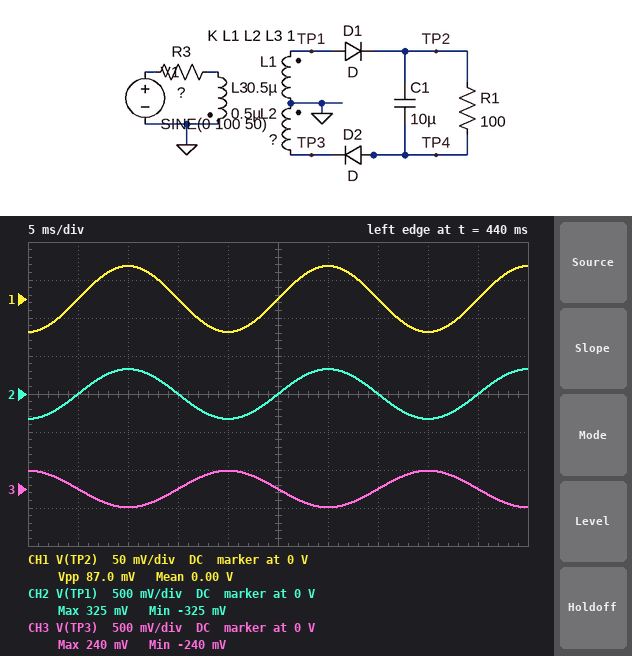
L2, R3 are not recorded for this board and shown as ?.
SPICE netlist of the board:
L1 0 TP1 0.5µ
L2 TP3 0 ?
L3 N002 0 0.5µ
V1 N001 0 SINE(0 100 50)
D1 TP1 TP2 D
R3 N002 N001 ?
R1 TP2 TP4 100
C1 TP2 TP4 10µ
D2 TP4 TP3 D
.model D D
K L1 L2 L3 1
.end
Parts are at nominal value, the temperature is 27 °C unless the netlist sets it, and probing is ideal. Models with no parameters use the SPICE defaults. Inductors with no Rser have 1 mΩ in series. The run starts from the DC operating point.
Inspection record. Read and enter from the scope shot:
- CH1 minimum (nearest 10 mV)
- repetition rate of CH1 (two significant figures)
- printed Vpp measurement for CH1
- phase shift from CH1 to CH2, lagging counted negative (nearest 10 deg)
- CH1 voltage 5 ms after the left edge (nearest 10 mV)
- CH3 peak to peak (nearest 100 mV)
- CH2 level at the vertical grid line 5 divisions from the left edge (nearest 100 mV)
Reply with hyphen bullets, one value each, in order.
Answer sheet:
- -40 mV
- 50 Hz
- 87.0 mV
- 0 deg
- 0 V
- 500 mV
- 0 V
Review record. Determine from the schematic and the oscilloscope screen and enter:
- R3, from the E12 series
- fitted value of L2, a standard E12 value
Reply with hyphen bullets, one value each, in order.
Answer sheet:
- 0.047 Ω
- 270 nH
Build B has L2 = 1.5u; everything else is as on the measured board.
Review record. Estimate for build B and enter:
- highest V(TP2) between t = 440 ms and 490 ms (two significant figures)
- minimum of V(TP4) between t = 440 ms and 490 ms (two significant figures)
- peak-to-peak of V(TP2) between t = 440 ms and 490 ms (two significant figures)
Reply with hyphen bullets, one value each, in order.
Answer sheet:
- 120 mV
- -120 mV
- 240 mV
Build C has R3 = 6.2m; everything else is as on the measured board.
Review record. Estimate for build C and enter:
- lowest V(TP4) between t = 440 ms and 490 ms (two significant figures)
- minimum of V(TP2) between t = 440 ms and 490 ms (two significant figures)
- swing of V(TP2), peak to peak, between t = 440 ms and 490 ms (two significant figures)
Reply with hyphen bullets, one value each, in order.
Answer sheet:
- -870 mV
- -290 mV
- 1.7 V
